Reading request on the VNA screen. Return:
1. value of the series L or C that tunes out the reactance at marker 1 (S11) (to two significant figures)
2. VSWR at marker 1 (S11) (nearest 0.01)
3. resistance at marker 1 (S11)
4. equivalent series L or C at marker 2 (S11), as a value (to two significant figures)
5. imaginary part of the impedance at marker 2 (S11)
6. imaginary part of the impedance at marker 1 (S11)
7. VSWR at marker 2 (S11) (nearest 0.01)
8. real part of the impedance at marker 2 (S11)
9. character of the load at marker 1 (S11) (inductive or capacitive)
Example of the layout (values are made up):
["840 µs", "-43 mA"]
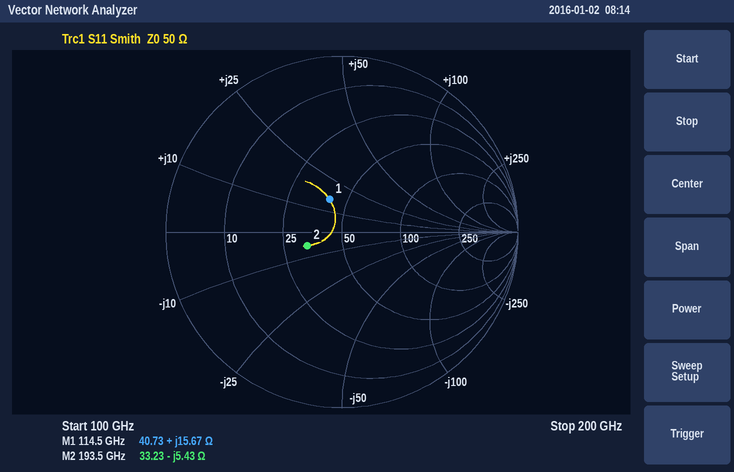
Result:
["89 fF", "1.49", "40.73 Ω", "150 fF", "-5.43 Ω", "+15.67 Ω", "1.54", "33.23 Ω", "inductive"]
